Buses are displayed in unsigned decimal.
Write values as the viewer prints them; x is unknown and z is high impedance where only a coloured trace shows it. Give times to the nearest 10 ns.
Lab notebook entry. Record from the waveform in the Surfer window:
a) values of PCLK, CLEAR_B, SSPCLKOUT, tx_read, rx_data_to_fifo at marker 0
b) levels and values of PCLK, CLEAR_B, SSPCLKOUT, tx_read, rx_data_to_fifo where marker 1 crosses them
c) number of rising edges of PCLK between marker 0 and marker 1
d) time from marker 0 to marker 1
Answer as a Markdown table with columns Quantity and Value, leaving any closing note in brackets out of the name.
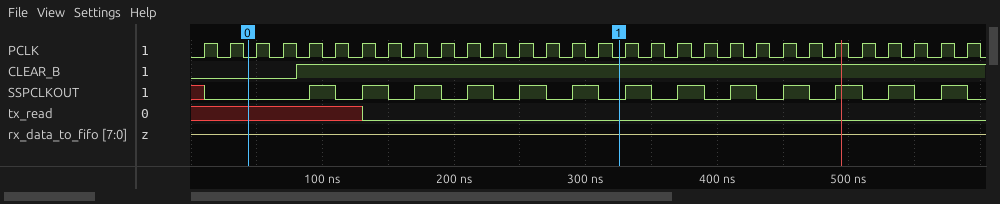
| Quantity | Value |
|---|---|
| values of PCLK, CLEAR_B, SSPCLKOUT, tx_read, rx_data_to_fifo at marker 0 | PCLK=0, CLEAR_B=0, SSPCLKOUT=0, tx_read=x, rx_data_to_fifo=z |
| levels and values of PCLK, CLEAR_B, SSPCLKOUT, tx_read, rx_data_to_fifo where marker 1 crosses them | PCLK=0, CLEAR_B=1, SSPCLKOUT=0, tx_read=0, rx_data_to_fifo=z |
| number of rising edges of PCLK between marker 0 and marker 1 | 14 |
| time from marker 0 to marker 1 | 280 ns |
